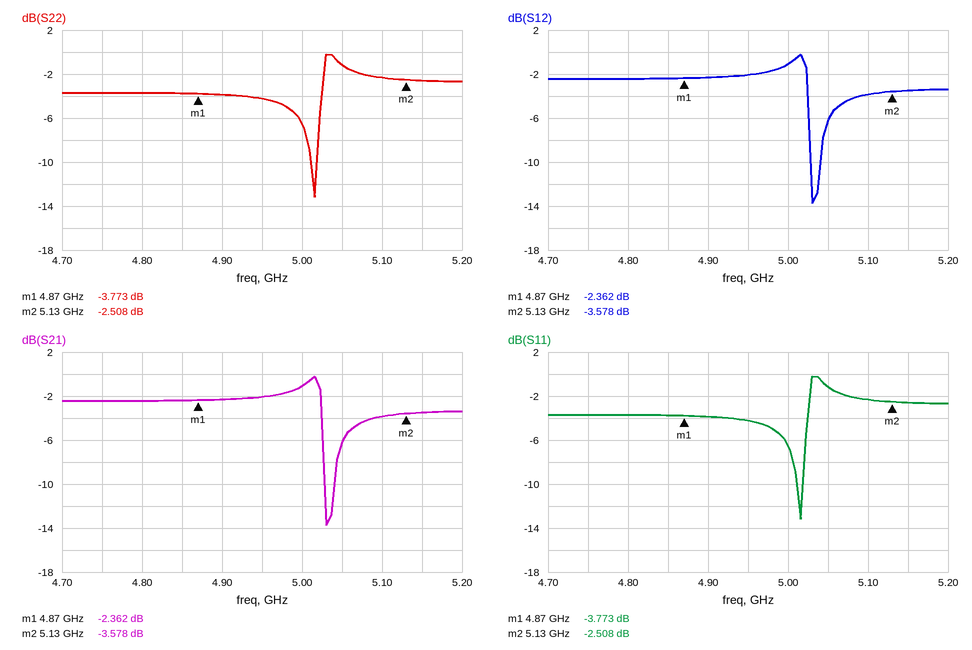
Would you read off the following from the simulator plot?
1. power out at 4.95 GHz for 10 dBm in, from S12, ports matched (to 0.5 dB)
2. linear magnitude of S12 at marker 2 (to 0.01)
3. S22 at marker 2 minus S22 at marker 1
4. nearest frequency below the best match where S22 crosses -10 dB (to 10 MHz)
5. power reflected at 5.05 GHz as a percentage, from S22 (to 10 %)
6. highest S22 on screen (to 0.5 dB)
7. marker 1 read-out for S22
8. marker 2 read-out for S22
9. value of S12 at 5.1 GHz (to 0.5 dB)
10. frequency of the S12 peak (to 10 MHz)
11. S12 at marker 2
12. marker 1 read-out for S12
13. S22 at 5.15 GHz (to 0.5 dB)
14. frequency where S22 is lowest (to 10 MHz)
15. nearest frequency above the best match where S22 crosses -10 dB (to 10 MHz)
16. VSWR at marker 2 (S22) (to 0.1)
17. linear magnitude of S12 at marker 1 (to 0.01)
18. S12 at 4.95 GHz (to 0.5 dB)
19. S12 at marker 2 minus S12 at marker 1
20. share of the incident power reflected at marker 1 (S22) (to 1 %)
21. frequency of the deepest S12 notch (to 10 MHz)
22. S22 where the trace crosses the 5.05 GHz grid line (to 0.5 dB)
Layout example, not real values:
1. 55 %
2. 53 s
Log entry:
1. 8.0 dBm
2. 0.66
3. 1.265 dB
4. 5.01 GHz
5. 80 %
6. 0.0 dB
7. -3.773 dB
8. -2.508 dB
9. -4.0 dB
10. 5.02 GHz
11. -3.578 dB
12. -2.362 dB
13. -2.5 dB
14. 5.02 GHz
15. 5.02 GHz
16. 7.0
17. 0.76
18. -2.0 dB
19. -1.216 dB
20. 42 %
21. 5.03 GHz
22. -1.0 dB
